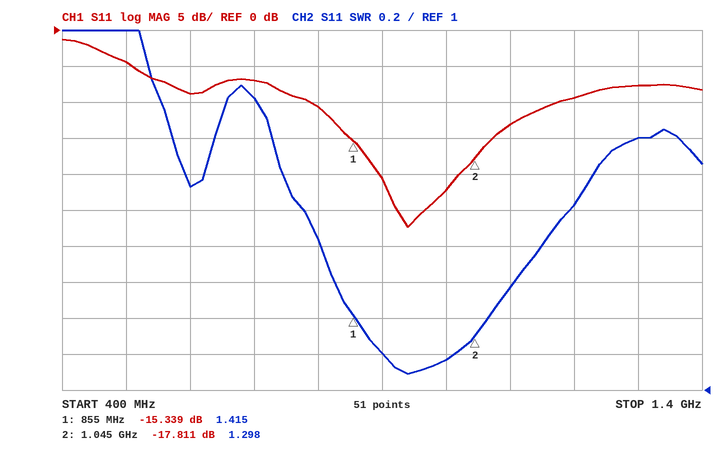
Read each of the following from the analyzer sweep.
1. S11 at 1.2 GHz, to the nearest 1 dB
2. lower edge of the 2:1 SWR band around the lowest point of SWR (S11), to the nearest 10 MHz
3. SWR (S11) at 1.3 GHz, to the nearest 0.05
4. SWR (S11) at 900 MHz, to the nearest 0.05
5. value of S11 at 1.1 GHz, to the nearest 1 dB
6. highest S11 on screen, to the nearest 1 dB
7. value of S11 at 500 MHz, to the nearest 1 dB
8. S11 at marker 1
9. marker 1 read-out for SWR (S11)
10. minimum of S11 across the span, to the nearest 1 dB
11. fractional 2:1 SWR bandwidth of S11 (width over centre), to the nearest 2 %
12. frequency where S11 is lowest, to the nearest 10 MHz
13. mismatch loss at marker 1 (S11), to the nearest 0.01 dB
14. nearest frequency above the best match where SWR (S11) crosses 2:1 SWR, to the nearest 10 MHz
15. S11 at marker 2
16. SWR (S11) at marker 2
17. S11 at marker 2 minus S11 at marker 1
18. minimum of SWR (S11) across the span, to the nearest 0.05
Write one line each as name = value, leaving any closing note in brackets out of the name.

S11 at 1.2 GHz, to the nearest 1 dB = -9 dB
lower edge of the 2:1 SWR band around the lowest point of SWR (S11), to the nearest 10 MHz = 780 MHz
SWR (S11) at 1.3 GHz, to the nearest 0.05 = 2.40
SWR (S11) at 900 MHz, to the nearest 0.05 = 1.20
value of S11 at 1.1 GHz, to the nearest 1 dB = -13 dB
highest S11 on screen, to the nearest 1 dB = -1 dB
value of S11 at 500 MHz, to the nearest 1 dB = -4 dB
S11 at marker 1 = -15.339 dB
marker 1 read-out for SWR = 1.415
minimum of S11 across the span, to the nearest 1 dB = -27 dB
fractional 2:1 SWR bandwidth of S11 (width over centre), to the nearest 2 % = 42 %
frequency where S11 is lowest, to the nearest 10 MHz = 940 MHz
mismatch loss at marker 1 (S11), to the nearest 0.01 dB = 0.13 dB
nearest frequency above the best match where SWR (S11) crosses 2:1 SWR, to the nearest 10 MHz = 1.19 GHz
S11 at marker 2 = -17.811 dB
SWR (S11) at marker 2 = 1.298
S11 at marker 2 minus S11 at marker 1 = -2.472 dB
minimum of SWR (S11) across the span, to the nearest 0.05 = 1.10
